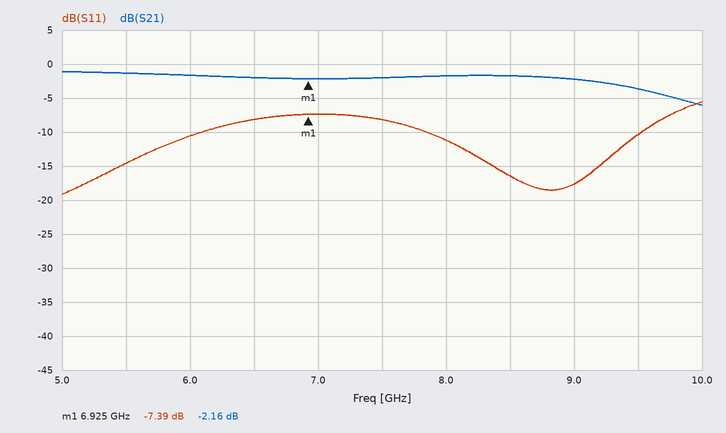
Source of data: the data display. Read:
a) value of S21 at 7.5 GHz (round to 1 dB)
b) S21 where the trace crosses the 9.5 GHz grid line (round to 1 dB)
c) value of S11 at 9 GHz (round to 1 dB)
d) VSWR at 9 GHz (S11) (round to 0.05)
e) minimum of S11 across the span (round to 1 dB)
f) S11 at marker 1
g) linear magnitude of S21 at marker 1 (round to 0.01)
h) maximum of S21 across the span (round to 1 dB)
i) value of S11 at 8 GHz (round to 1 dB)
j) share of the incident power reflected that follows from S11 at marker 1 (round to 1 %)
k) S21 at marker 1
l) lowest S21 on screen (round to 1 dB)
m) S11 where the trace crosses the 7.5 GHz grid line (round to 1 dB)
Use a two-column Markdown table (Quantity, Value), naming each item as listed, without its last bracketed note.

| Quantity | Value |
|---|---|
| value of S21 at 7.5 GHz | -2 dB |
| S21 where the trace crosses the 9.5 GHz grid line | -4 dB |
| value of S11 at 9 GHz | -18 dB |
| VSWR at 9 GHz (S11) | 1.30 |
| minimum of S11 across the span | -19 dB |
| S11 at marker 1 | -7.39 dB |
| linear magnitude of S21 at marker 1 | 0.78 |
| maximum of S21 across the span | -1 dB |
| value of S11 at 8 GHz | -11 dB |
| share of the incident power reflected that follows from S11 at marker 1 | 18 % |
| S21 at marker 1 | -2.16 dB |
| lowest S21 on screen | -6 dB |
| S11 where the trace crosses the 7.5 GHz grid line | -8 dB |
